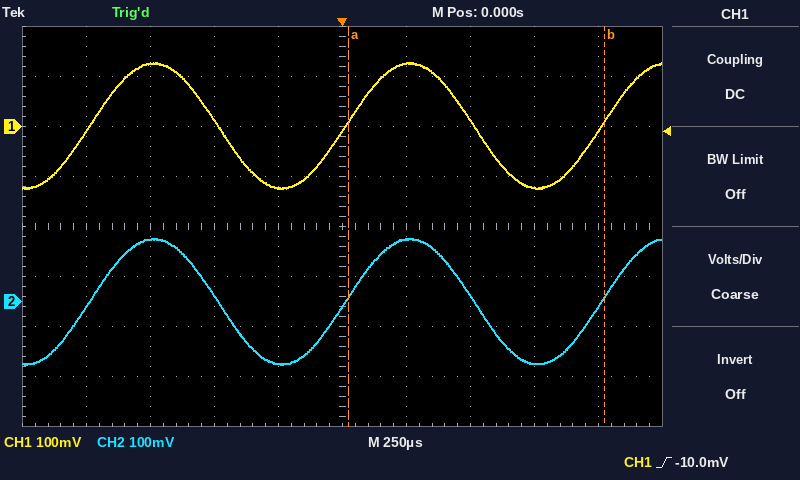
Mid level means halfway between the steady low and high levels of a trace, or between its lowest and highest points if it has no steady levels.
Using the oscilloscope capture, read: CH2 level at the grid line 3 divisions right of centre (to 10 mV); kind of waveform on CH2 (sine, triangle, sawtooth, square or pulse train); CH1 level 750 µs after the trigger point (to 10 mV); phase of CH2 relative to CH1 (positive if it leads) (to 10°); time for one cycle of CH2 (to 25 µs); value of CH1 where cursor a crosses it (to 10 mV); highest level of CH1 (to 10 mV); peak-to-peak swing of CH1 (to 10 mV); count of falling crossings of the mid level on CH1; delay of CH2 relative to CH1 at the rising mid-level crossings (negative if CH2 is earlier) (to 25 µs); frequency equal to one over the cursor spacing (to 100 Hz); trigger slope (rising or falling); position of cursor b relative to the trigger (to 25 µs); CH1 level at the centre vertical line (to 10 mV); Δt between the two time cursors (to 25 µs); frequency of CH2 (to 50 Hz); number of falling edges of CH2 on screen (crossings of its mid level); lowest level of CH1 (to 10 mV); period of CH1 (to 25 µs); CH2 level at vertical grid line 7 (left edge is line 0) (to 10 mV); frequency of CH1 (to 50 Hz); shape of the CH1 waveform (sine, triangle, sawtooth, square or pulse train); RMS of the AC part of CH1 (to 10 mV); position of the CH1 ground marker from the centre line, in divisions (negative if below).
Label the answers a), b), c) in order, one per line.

a) -120 mV
b) sine
c) -120 mV
d) 0°
e) 1.000 ms
f) 10 mV
g) 130 mV
h) 250 mV
i) 2
j) 0 µs
k) 1.0 kHz
l) rising
m) +1.025 ms
n) -10 mV
o) 1.000 ms
p) 1.00 kHz
q) 2
r) -120 mV
s) 1.000 ms
t) 10 mV
u) 1.00 kHz
v) sine
w) 90 mV
x) +2.0 div
